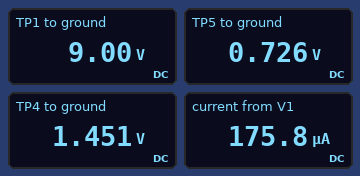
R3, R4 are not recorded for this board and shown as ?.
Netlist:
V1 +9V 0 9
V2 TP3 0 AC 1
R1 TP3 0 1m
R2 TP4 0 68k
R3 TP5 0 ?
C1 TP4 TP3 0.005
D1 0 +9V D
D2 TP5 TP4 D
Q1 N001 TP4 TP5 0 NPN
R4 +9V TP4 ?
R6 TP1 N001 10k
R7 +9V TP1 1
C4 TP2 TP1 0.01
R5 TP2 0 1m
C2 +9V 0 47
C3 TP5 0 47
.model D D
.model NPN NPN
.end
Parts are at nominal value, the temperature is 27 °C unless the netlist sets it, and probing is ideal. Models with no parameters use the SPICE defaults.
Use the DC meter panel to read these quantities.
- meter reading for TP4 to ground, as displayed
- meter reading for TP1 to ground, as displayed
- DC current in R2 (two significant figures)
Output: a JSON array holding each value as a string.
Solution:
["1.451 V", "9.00 V", "21 µA"]
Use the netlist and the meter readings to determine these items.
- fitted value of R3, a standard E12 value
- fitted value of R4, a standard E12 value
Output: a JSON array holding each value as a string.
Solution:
["4.7 kΩ", "330 kΩ"]
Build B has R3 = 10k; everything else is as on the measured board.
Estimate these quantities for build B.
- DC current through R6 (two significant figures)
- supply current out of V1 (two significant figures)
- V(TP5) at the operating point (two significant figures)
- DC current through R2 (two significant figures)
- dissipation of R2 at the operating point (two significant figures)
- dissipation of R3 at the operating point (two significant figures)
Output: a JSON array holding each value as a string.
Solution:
["78 µA", "100 µA", "790 mV", "22 µA", "33 µW", "62 µW"]
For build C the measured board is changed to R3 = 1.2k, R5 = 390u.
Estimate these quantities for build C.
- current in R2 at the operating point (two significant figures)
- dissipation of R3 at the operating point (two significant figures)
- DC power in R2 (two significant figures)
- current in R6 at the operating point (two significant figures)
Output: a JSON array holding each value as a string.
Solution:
["19 µA", "240 µW", "24 µW", "440 µA"]
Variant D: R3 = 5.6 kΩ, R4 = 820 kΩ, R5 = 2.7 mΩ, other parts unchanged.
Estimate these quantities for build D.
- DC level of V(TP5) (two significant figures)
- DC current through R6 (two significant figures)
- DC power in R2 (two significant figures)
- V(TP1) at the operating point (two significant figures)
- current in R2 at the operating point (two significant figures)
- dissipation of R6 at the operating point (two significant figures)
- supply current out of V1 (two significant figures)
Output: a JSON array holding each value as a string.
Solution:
["39 mV", "6.9 µA", "6.9 µW", "9.0 V", "10 µA", "480 nW", "17 µA"]
